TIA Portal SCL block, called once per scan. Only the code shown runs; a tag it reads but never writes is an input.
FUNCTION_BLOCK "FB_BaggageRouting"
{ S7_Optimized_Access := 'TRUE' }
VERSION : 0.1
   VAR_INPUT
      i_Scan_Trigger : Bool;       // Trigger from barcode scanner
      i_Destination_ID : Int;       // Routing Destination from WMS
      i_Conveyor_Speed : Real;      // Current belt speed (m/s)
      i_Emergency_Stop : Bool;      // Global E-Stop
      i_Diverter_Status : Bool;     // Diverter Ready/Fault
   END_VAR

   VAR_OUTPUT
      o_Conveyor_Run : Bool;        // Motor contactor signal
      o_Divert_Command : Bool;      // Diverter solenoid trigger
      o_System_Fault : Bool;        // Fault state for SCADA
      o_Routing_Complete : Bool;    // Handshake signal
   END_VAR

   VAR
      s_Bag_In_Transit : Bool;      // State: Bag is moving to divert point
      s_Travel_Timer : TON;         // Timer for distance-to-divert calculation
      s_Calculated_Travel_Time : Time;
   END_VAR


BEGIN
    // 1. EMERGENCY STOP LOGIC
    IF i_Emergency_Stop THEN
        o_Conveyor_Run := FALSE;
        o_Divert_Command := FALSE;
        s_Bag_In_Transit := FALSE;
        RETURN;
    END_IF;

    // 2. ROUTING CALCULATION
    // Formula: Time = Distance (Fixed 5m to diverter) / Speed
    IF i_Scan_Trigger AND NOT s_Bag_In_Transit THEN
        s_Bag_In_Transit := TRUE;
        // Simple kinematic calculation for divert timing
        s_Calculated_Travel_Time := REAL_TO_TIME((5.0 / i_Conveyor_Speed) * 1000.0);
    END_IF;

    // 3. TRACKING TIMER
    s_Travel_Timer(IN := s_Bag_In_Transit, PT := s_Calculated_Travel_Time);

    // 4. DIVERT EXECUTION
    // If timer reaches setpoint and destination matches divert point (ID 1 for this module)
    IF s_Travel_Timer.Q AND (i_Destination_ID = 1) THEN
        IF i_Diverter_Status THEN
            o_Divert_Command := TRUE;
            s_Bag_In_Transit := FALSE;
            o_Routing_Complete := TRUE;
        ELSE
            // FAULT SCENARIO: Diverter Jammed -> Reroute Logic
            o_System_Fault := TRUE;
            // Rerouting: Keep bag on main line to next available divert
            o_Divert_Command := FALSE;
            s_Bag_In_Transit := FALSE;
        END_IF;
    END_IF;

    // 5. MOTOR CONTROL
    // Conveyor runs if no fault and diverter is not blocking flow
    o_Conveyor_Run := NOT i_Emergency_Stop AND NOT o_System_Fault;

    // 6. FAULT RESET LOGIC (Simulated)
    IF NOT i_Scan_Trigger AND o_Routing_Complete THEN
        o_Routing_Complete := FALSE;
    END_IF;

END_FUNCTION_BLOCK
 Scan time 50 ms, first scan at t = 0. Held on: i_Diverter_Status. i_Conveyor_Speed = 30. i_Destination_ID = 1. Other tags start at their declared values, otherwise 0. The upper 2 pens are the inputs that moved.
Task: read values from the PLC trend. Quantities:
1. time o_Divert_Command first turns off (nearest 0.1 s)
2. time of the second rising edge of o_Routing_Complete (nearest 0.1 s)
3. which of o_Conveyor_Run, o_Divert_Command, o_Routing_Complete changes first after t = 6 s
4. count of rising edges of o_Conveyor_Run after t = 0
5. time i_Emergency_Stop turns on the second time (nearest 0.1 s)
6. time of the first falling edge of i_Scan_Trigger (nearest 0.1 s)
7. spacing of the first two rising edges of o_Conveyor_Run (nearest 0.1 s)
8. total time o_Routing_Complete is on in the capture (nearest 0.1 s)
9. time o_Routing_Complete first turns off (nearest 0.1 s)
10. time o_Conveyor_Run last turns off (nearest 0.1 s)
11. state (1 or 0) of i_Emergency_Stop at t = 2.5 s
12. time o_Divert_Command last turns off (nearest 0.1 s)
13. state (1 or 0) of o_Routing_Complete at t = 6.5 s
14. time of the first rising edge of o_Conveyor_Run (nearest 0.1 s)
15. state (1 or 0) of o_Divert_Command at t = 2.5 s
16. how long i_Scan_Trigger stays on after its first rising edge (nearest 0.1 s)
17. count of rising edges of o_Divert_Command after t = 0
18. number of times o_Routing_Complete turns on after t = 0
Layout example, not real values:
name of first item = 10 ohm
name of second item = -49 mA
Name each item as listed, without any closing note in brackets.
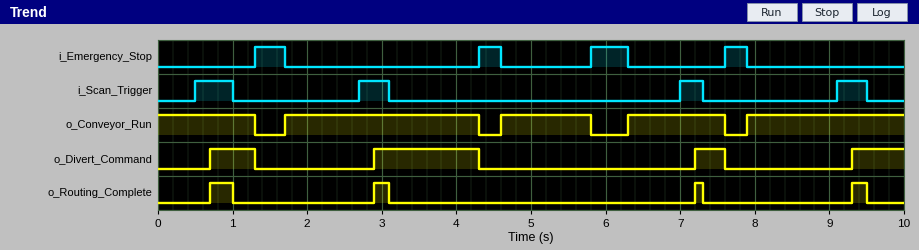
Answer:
time o_Divert_Command first turns off = 1.3 s
time of the second rising edge of o_Routing_Complete = 2.9 s
which of o_Conveyor_Run, o_Divert_Command, o_Routing_Complete changes first after t = 6 s = o_Conveyor_Run
count of rising edges of o_Conveyor_Run after t = 0 = 4
time i_Emergency_Stop turns on the second time = 4.3 s
time of the first falling edge of i_Scan_Trigger = 1.0 s
spacing of the first two rising edges of o_Conveyor_Run = 2.9 s
total time o_Routing_Complete is on in the capture = 0.8 s
time o_Routing_Complete first turns off = 1.0 s
time o_Conveyor_Run last turns off = 7.6 s
state (1 or 0) of i_Emergency_Stop at t = 2.5 s = 0
time o_Divert_Command last turns off = 7.6 s
state (1 or 0) of o_Routing_Complete at t = 6.5 s = 0
time of the first rising edge of o_Conveyor_Run = 1.7 s
state (1 or 0) of o_Divert_Command at t = 2.5 s = 0
how long i_Scan_Trigger stays on after its first rising edge = 0.5 s
count of rising edges of o_Divert_Command after t = 0 = 4
number of times o_Routing_Complete turns on after t = 0 = 4
